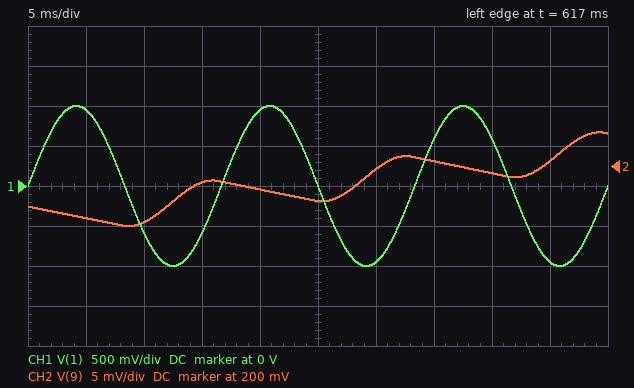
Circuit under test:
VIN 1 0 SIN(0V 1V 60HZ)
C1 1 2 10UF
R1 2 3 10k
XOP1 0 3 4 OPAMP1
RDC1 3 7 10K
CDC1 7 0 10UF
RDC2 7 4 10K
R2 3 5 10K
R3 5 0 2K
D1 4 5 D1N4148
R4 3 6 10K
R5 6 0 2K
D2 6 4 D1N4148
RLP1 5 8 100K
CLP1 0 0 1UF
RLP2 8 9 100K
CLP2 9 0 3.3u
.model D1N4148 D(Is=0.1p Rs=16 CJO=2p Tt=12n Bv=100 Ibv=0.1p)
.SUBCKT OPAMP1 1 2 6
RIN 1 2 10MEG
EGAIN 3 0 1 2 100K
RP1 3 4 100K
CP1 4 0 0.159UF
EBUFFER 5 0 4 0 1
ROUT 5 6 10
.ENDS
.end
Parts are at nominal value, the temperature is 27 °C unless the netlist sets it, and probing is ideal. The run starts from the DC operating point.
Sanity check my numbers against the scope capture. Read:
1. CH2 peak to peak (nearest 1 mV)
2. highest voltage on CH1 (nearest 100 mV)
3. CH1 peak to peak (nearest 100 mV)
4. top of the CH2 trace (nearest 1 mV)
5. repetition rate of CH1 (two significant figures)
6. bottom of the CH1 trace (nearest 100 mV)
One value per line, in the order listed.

12 mV
1.0 V
2.0 V
204 mV
60 Hz
-1.0 V
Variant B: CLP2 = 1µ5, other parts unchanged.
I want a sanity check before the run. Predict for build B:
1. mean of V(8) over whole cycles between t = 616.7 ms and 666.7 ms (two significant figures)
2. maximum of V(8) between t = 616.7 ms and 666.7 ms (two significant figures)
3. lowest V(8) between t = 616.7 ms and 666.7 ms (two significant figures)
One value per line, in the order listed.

300 mV
640 mV
140 mV
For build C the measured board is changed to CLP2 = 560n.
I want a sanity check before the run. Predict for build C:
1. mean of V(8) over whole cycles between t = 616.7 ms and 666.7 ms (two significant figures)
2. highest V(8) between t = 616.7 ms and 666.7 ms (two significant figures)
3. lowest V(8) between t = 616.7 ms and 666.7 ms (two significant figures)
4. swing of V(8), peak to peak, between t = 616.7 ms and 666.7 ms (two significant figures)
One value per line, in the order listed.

320 mV
660 mV
150 mV
500 mV
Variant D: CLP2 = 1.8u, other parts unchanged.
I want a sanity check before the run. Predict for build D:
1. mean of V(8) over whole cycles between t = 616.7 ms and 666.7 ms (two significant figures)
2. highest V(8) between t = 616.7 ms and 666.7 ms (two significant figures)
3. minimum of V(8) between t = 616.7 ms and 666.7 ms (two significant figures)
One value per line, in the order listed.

290 mV
630 mV
130 mV
